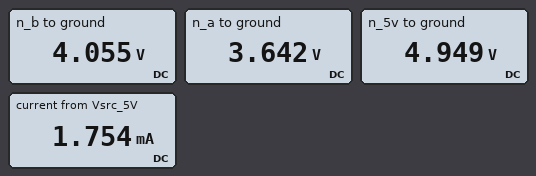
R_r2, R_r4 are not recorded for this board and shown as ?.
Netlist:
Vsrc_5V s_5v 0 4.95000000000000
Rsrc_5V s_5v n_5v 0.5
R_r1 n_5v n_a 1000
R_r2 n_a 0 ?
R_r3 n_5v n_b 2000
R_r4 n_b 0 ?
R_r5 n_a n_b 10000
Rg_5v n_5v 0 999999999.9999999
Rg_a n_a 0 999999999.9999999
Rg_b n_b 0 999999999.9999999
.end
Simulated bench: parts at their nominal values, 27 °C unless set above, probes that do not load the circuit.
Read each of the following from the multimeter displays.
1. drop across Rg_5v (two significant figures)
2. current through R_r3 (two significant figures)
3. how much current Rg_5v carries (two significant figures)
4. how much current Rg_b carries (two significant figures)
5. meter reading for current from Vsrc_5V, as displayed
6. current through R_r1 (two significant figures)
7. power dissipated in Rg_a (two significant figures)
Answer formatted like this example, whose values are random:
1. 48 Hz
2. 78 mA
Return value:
1. 4.9 V
2. 450 µA
3. 4.9 nA
4. 4.1 nA
5. 1.754 mA
6. 1.3 mA
7. 13 nW
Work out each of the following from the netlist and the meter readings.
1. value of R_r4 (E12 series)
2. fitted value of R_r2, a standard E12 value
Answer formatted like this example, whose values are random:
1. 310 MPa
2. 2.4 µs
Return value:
1. 10 kΩ
2. 2.7 kΩ
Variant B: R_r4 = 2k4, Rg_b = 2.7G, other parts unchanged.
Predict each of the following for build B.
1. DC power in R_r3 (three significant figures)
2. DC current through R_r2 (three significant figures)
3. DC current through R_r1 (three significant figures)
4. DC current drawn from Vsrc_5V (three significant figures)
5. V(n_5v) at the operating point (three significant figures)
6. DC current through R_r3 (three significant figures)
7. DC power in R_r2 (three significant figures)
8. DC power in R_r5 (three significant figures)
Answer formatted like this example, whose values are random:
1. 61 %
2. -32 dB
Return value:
1. 2.34 mW
2. 1.32 mA
3. 1.39 mA
4. 2.48 mA
5. 4.95 V
6. 1.08 mA
7. 4.68 mW
8. 59.5 µW
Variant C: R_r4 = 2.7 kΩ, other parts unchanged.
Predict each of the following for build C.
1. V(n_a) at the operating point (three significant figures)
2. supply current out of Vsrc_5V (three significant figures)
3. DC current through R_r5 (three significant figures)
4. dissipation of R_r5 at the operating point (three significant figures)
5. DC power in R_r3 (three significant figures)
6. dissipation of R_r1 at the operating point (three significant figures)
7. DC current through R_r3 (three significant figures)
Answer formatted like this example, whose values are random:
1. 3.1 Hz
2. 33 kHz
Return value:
1. 3.56 V
2. 2.40 mA
3. 64.7 µA
4. 41.8 µW
5. 2.06 mW
6. 1.92 mW
7. 1.02 mA
